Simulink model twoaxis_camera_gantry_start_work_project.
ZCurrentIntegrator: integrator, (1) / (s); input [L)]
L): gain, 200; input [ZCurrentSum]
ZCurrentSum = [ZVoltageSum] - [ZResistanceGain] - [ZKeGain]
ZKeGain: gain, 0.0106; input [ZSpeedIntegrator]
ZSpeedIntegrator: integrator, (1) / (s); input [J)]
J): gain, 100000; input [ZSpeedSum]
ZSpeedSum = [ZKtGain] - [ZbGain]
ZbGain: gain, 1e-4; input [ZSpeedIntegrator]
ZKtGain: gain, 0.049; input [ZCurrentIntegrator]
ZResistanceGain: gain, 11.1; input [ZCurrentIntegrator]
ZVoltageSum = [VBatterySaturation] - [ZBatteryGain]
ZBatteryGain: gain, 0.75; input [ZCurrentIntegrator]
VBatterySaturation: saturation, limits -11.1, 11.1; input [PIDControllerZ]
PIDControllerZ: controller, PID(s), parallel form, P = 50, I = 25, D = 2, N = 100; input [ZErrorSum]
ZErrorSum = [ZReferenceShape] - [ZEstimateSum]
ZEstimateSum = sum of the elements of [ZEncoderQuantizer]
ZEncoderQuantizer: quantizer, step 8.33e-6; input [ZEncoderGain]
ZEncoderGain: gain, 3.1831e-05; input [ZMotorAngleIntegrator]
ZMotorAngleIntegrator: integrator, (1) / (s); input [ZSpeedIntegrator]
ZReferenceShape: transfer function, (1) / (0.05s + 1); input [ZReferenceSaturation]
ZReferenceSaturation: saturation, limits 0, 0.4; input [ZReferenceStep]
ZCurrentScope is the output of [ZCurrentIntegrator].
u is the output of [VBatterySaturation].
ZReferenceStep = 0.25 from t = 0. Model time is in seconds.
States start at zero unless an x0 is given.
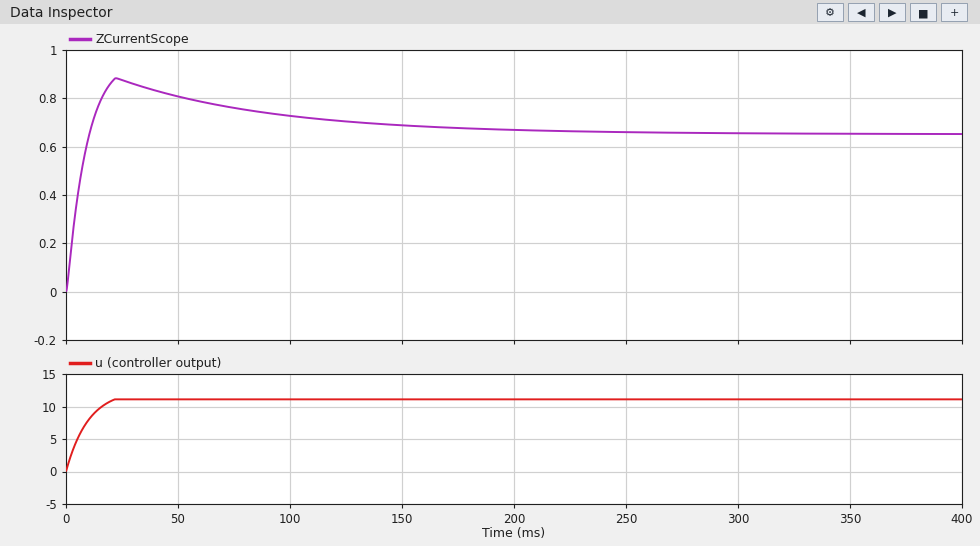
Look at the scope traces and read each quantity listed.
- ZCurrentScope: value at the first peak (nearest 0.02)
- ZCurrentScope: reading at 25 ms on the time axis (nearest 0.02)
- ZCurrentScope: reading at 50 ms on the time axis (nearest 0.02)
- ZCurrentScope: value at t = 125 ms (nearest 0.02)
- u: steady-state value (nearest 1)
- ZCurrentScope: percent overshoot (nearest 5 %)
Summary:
0.88
0.88
0.80
0.70
11
35 %
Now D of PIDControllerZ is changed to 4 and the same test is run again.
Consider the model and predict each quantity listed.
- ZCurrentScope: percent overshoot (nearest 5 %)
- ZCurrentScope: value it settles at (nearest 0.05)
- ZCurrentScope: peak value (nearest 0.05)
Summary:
40 %
0.65
0.90
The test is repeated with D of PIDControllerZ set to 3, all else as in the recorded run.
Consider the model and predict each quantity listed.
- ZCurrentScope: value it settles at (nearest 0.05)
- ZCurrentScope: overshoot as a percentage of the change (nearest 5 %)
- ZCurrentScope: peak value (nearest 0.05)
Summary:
0.65
40 %
0.90
